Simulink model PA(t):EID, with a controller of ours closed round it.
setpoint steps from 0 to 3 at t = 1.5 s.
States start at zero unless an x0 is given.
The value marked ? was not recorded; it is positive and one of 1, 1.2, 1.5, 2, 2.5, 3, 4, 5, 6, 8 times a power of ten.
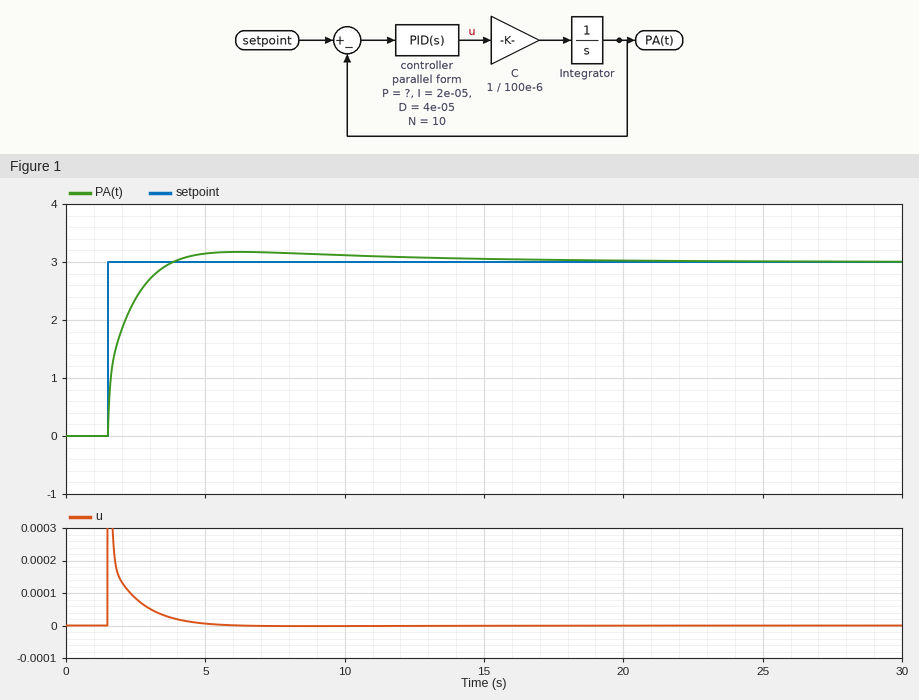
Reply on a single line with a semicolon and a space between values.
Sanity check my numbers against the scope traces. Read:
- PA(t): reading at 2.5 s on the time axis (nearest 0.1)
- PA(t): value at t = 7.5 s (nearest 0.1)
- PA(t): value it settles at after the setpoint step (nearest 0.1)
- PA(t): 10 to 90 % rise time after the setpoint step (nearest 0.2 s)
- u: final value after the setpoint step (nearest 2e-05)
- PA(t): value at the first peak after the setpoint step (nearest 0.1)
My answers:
2.4; 3.2; 3.0; 1.4 s; 0.00000; 3.2
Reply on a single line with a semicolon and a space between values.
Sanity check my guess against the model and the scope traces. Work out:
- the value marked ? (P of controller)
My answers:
0.00015
